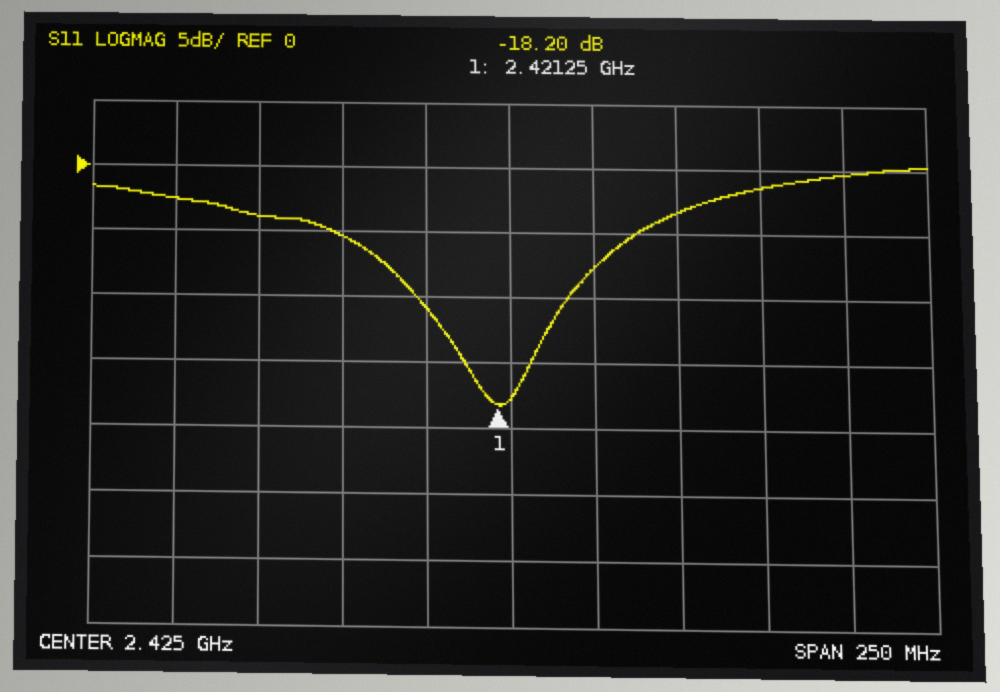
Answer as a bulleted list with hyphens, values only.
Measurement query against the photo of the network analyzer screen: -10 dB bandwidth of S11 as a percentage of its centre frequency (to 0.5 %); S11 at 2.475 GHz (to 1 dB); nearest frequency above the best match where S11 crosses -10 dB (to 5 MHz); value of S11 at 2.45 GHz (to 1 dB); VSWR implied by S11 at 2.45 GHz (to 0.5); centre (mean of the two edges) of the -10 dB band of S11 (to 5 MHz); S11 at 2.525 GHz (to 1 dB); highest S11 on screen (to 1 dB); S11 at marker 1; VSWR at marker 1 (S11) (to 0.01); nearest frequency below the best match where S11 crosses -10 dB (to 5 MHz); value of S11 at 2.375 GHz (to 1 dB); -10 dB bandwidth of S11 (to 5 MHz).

- 2.0 %
- -3 dB
- 2.440 GHz
- -8 dB
- 2.5
- 2.420 GHz
- 0 dB
- 0 dB
- -18.20 dB
- 1.28
- 2.395 GHz
- -5 dB
- 45 MHz
